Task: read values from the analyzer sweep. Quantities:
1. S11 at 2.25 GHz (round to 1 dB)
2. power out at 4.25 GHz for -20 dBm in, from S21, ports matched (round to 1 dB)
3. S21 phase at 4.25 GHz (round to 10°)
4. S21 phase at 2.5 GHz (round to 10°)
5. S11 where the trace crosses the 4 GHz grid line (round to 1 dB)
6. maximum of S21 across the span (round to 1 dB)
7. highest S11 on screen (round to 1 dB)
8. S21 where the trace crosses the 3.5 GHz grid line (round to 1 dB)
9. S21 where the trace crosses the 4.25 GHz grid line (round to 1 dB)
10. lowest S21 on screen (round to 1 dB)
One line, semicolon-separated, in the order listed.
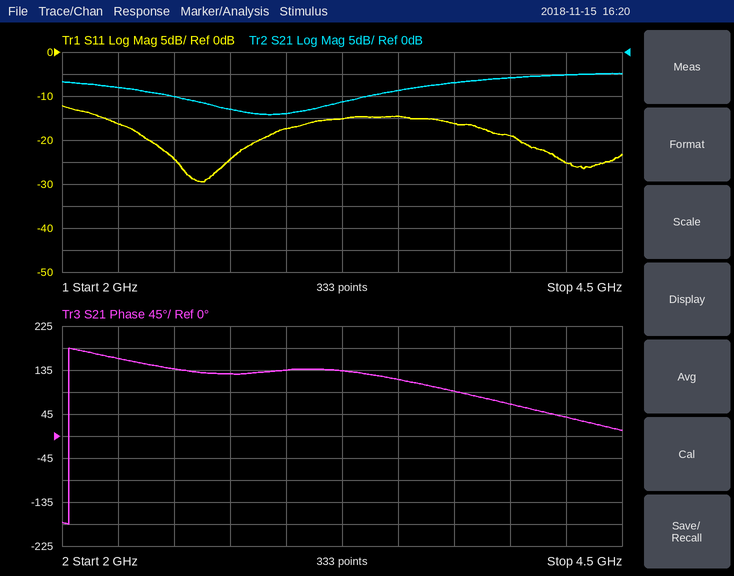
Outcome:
-16 dB; -25 dBm; 40°; 140°; -19 dB; -5 dB; -12 dB; -9 dB; -5 dB; -14 dB
